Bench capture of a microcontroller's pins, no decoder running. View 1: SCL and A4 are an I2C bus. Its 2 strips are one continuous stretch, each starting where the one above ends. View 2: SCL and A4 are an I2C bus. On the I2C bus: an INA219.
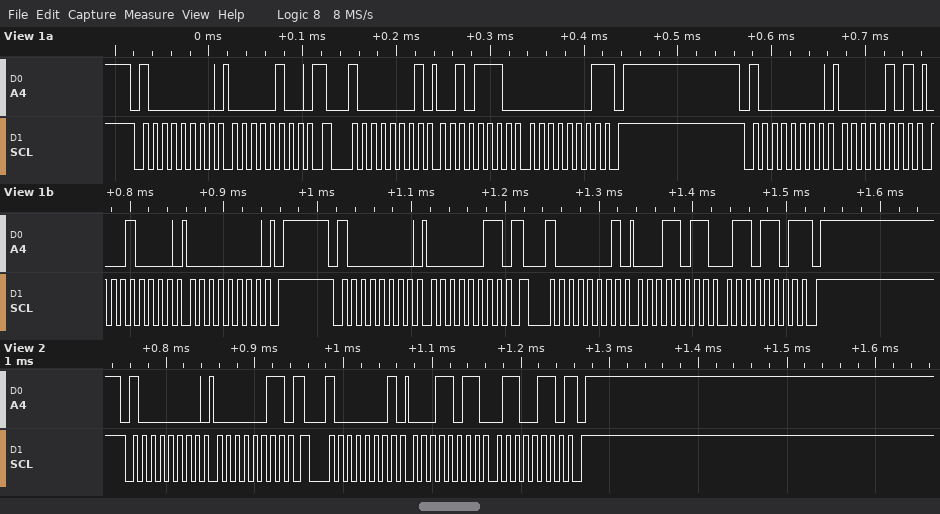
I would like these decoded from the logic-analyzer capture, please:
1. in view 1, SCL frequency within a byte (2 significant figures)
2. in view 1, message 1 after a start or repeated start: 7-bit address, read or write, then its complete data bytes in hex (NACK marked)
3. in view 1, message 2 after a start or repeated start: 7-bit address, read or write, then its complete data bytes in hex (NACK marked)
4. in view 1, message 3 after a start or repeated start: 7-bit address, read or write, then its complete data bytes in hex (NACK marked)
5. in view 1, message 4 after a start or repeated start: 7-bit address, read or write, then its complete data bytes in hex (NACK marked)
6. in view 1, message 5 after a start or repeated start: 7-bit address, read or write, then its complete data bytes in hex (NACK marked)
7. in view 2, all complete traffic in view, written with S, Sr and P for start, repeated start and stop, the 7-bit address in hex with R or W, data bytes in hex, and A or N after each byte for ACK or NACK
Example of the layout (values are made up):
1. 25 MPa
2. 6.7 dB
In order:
1. 100 kHz
2. 0x40 write: 04
3. 0x40 read: 2E 01 NACK
4. 0x40 write: 05 10 00
5. 0x40 write: 03
6. 0x40 read: 1B 6D NACK
7. S 40W A 03 A Sr 40R A 1B A 66 N P
